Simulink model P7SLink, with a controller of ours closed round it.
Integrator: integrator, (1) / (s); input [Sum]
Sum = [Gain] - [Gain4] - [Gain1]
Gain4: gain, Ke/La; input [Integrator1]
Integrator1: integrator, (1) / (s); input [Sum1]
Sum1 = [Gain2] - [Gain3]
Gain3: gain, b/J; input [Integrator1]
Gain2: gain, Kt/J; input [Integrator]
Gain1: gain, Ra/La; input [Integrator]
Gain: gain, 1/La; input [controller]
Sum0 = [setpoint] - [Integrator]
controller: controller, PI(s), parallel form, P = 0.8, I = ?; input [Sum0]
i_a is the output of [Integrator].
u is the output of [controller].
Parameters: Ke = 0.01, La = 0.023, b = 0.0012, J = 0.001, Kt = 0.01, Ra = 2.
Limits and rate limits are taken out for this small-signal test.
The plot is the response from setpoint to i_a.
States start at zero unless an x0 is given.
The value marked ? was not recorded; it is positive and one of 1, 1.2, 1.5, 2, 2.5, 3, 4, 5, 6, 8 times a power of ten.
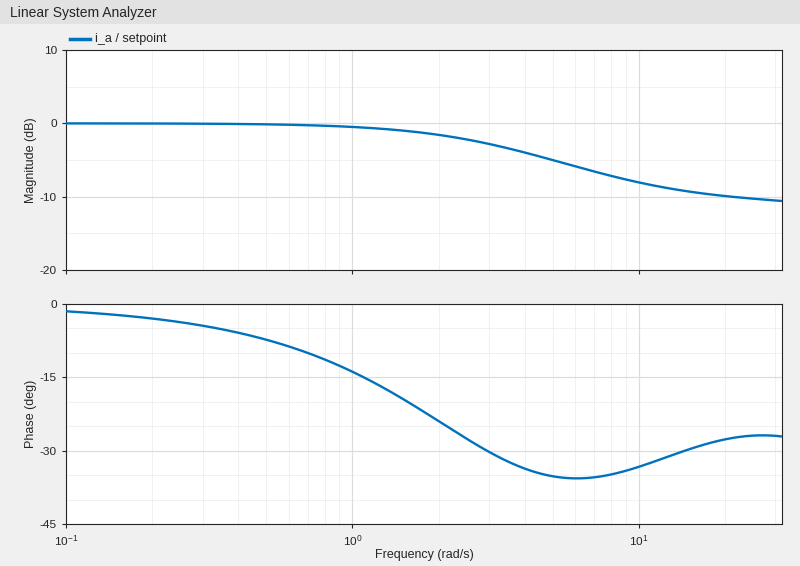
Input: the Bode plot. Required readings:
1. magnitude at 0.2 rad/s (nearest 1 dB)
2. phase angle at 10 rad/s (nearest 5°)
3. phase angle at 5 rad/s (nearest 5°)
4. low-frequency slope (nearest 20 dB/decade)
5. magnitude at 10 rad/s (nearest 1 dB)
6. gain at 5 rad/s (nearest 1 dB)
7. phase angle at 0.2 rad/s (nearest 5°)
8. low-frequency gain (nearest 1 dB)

0 dB
-35°
-35°
0 dB/decade
-8 dB
-5 dB
-5°
0 dB
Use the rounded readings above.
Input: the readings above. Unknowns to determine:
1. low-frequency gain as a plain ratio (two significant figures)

1.0
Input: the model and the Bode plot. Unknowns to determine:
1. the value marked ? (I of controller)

8
